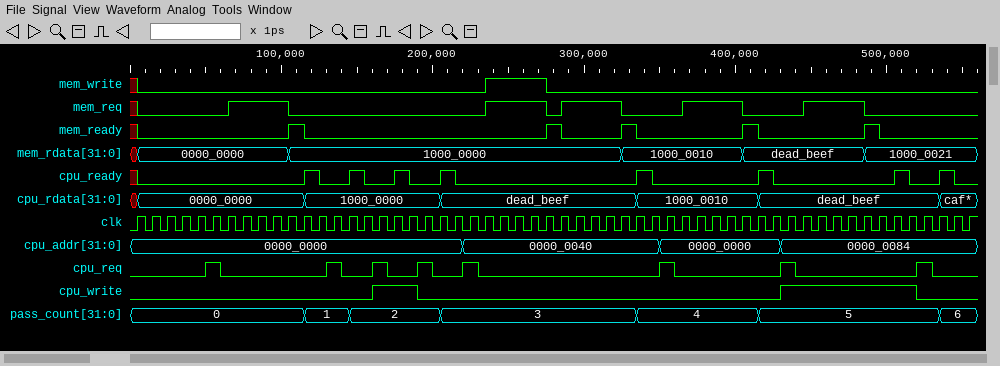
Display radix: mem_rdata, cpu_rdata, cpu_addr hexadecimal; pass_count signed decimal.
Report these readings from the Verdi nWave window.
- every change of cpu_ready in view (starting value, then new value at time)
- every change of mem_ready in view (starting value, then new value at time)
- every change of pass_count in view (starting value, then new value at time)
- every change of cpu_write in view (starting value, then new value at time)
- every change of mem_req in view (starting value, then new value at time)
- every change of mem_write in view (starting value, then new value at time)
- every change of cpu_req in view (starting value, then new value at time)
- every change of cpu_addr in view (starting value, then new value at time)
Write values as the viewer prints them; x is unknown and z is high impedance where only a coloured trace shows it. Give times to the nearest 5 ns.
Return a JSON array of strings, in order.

["x, 0 at 5 ns, 1 at 115 ns, 0 at 125 ns, 1 at 145 ns, 0 at 155 ns, 1 at 175 ns, 0 at 185 ns, 1 at 205 ns, 0 at 215 ns, 1 at 335 ns, 0 at 345 ns, 1 at 415 ns, 0 at 425 ns, 1 at 505 ns, 0 at 515 ns, 1 at 535 ns, 0 at 545 ns", "x, 0 at 5 ns, 1 at 105 ns, 0 at 115 ns, 1 at 275 ns, 0 at 285 ns, 1 at 325 ns, 0 at 335 ns, 1 at 405 ns, 0 at 415 ns, 1 at 485 ns, 0 at 495 ns", "0, 1 at 115 ns, 2 at 145 ns, 3 at 205 ns, 4 at 335 ns, 5 at 415 ns, 6 at 535 ns", "0, 1 at 160 ns, 0 at 190 ns, 1 at 430 ns, 0 at 520 ns", "x, 0 at 5 ns, 1 at 65 ns, 0 at 105 ns, 1 at 235 ns, 0 at 275 ns, 1 at 285 ns, 0 at 325 ns, 1 at 365 ns, 0 at 405 ns, 1 at 445 ns, 0 at 485 ns", "x, 0 at 5 ns, 1 at 235 ns, 0 at 275 ns", "0, 1 at 50 ns, 0 at 60 ns, 1 at 130 ns, 0 at 140 ns, 1 at 160 ns, 0 at 170 ns, 1 at 190 ns, 0 at 200 ns, 1 at 220 ns, 0 at 230 ns, 1 at 350 ns, 0 at 360 ns, 1 at 430 ns, 0 at 440 ns, 1 at 520 ns, 0 at 530 ns", "0000_0000, 0000_0040 at 220 ns, 0000_0000 at 350 ns, 0000_0084 at 430 ns"]
